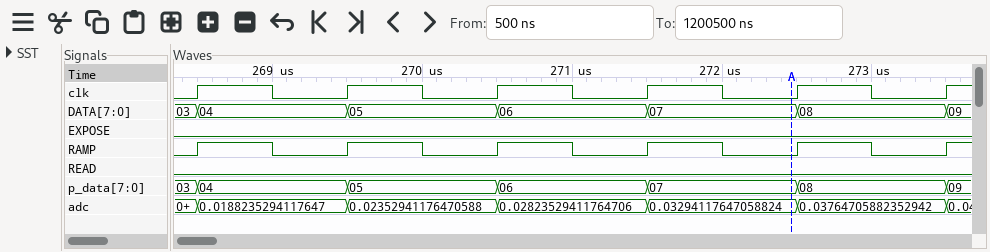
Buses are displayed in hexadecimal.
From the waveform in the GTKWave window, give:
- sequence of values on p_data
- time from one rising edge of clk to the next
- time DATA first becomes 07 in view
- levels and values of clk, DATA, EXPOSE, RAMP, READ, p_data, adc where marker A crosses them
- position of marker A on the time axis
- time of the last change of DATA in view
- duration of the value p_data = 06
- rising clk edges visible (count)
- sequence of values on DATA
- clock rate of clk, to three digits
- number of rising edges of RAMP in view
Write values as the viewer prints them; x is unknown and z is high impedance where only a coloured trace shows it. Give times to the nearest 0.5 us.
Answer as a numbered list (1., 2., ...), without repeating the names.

1. 03, 04, 05, 06, 07, 08, 09
2. 1 us
3. 271.5 us
4. clk=0, DATA=07, EXPOSE=0, RAMP=0, READ=0, p_data=07, adc=0.03294117647058824
5. 272.5 us
6. 273.5 us
7. 1 us
8. 6
9. 03, 04, 05, 06, 07, 08, 09
10. 1.00 MHz
11. 6
